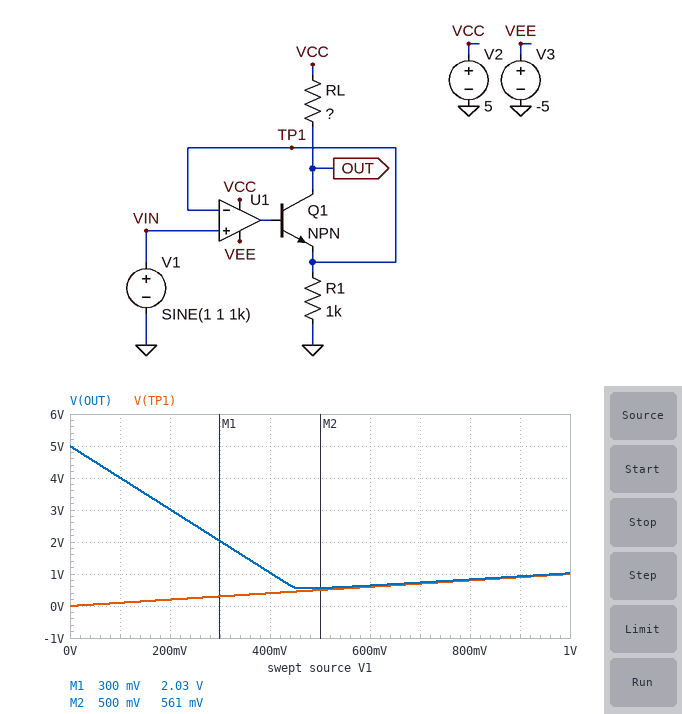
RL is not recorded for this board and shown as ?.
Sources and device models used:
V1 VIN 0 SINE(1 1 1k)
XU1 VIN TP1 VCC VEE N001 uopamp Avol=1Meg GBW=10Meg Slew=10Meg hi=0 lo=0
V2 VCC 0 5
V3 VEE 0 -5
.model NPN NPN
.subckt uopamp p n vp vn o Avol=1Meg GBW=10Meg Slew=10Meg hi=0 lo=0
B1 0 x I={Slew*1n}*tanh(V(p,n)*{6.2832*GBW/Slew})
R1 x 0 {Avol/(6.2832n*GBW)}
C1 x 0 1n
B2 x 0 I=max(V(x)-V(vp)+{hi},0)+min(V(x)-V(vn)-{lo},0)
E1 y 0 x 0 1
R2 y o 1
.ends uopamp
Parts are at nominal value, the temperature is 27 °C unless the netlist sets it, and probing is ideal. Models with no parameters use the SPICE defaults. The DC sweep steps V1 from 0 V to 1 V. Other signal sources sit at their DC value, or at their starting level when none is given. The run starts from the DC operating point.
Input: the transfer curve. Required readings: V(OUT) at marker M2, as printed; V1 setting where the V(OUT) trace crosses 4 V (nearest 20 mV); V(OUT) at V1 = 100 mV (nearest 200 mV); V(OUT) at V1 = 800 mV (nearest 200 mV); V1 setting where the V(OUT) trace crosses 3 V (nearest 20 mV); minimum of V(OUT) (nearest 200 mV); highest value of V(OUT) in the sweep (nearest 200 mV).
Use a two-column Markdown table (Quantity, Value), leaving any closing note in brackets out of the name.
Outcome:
| Quantity | Value |
|---|---|
| V(OUT) at marker M2, as printed | 561 mV |
| V1 setting where the V(OUT) trace crosses 4 V | 100 mV |
| V(OUT) at V1 = 100 mV | 4.0 V |
| V(OUT) at V1 = 800 mV | 800 mV |
| V1 setting where the V(OUT) trace crosses 3 V | 200 mV |
| minimum of V(OUT) | 600 mV |
| highest value of V(OUT) in the sweep | 5.0 V |
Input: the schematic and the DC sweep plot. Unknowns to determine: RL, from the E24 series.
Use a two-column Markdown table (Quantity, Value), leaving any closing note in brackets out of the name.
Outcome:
| Quantity | Value |
|---|---|
| RL, from the E24 series | 10 kΩ |
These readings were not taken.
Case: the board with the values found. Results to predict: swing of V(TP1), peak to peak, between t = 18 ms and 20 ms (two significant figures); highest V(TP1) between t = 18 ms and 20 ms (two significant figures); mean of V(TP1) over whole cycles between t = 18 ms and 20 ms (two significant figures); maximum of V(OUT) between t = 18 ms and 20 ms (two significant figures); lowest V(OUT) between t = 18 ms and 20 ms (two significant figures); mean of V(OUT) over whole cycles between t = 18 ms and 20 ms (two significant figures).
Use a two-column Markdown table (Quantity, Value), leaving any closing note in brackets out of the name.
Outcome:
| Quantity | Value |
|---|---|
| swing of V(TP1), peak to peak, between t = 18 ms and 20 ms | 2.0 V |
| highest V(TP1) between t = 18 ms and 20 ms | 2.0 V |
| mean of V(TP1) over whole cycles between t = 18 ms and 20 ms | 1.0 V |
| maximum of V(OUT) between t = 18 ms and 20 ms | 5.0 V |
| lowest V(OUT) between t = 18 ms and 20 ms | 550 mV |
| mean of V(OUT) over whole cycles between t = 18 ms and 20 ms | 2.1 V |
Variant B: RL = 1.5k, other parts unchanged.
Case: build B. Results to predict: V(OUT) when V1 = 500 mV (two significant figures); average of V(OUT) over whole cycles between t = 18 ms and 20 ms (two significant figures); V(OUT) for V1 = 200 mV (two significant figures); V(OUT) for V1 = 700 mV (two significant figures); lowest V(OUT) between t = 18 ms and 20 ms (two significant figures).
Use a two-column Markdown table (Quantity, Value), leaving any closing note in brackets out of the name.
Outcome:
| Quantity | Value |
|---|---|
| V(OUT) when V1 = 500 mV | 4.3 V |
| average of V(OUT) over whole cycles between t = 18 ms and 20 ms | 3.5 V |
| V(OUT) for V1 = 200 mV | 4.7 V |
| V(OUT) for V1 = 700 mV | 4.0 V |
| lowest V(OUT) between t = 18 ms and 20 ms | 2.1 V |
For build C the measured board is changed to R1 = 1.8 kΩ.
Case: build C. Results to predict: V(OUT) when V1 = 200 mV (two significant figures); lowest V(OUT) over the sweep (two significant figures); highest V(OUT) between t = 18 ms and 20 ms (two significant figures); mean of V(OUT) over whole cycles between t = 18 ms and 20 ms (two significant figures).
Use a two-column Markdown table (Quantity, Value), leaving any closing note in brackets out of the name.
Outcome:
| Quantity | Value |
|---|---|
| V(OUT) when V1 = 200 mV | 3.9 V |
| lowest V(OUT) over the sweep | 870 mV |
| highest V(OUT) between t = 18 ms and 20 ms | 5.0 V |
| mean of V(OUT) over whole cycles between t = 18 ms and 20 ms | 2.4 V |
